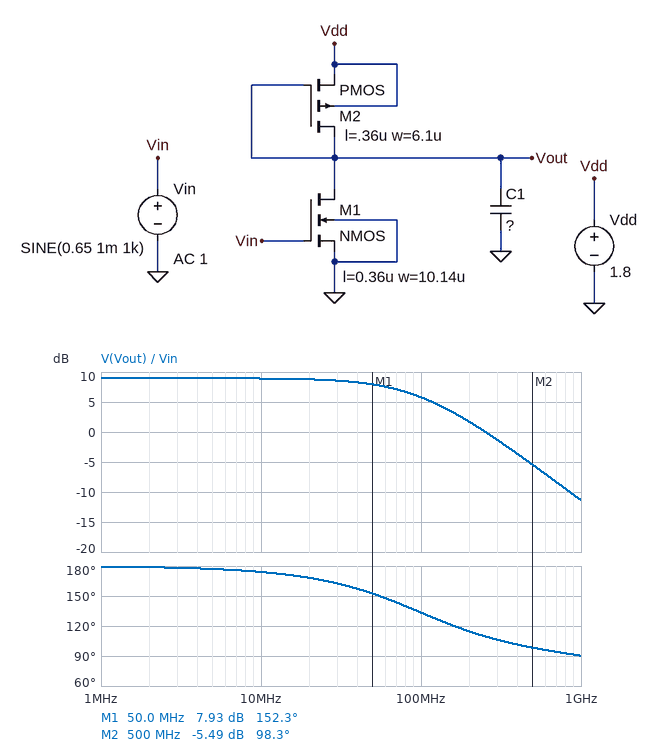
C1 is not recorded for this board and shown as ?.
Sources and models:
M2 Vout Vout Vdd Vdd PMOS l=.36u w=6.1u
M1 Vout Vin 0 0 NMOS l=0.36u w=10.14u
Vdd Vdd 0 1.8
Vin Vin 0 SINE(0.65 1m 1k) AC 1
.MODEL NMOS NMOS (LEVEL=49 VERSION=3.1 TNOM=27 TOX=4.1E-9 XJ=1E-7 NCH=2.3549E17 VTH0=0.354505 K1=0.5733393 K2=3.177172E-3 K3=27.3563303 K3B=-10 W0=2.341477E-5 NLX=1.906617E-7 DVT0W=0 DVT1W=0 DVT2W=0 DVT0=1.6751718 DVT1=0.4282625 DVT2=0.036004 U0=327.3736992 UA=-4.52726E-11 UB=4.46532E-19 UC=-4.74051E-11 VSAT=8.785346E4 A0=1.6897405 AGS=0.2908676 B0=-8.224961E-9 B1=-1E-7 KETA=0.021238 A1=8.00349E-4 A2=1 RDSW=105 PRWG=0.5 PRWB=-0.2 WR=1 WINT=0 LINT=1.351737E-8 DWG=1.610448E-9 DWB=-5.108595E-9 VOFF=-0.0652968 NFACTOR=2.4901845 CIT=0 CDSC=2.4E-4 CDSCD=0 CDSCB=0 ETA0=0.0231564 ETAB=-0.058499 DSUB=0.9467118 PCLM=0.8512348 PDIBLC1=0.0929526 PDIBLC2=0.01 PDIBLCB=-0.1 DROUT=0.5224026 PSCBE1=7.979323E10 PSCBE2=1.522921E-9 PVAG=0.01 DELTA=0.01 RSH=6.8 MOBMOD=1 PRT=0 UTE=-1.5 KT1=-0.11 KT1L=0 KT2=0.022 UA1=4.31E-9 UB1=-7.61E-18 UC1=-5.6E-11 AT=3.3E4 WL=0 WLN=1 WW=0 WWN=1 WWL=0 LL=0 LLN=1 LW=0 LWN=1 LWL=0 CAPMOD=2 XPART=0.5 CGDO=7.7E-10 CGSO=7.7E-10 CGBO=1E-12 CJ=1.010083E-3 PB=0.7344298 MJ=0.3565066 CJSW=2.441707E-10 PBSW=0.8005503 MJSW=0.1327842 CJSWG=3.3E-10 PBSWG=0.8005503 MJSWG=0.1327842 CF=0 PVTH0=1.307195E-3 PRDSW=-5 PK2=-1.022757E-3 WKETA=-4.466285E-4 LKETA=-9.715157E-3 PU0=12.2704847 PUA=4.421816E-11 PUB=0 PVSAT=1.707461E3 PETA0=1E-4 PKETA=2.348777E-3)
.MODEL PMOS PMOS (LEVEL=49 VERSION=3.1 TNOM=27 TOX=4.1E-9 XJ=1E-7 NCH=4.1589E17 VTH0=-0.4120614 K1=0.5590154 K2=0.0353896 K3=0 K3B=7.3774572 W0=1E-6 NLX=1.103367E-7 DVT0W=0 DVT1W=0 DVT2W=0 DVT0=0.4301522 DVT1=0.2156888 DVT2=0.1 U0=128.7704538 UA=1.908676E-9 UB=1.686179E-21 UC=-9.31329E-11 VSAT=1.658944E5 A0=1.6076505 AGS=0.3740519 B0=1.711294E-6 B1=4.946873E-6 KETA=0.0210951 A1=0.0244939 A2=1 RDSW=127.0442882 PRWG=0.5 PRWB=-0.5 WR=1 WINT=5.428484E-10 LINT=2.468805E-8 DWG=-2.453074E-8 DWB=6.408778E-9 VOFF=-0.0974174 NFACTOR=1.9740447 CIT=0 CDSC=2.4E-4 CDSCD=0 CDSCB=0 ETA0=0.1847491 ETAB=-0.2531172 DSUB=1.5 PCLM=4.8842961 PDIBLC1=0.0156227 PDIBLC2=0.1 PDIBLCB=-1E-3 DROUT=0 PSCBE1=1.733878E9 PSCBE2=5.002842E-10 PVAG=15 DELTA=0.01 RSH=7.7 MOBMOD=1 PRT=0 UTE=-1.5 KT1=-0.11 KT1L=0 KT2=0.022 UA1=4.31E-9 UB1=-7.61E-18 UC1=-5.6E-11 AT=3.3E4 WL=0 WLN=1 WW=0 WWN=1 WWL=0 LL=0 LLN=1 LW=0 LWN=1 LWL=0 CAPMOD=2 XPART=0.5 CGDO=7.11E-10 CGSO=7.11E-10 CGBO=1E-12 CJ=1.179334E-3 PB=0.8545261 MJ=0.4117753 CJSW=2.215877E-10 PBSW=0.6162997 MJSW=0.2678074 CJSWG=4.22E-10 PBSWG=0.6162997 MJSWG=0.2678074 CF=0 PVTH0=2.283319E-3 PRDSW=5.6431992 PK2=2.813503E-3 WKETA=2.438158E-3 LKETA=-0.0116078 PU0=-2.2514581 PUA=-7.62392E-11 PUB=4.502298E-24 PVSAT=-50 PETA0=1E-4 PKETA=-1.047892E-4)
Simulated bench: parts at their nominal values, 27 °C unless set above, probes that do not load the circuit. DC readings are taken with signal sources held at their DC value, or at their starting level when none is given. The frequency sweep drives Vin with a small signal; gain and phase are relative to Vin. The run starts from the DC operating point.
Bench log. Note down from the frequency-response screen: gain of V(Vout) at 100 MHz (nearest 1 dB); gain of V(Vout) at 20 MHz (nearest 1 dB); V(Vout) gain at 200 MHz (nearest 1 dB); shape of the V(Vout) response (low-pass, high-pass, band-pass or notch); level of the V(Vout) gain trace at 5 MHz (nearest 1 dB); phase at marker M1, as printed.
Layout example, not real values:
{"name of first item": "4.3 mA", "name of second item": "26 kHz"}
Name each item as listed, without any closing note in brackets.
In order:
{"gain of V(Vout) at 100 MHz": "6 dB", "gain of V(Vout) at 20 MHz": "9 dB", "V(Vout) gain at 200 MHz": "2 dB", "shape of the V(Vout) response": "low-pass", "level of the V(Vout) gain trace at 5 MHz": "9 dB", "phase at marker M1, as printed": "152.3 deg"}
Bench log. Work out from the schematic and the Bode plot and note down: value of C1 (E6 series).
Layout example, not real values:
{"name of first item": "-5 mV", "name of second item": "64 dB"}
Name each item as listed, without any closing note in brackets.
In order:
{"value of C1": "680 fF"}
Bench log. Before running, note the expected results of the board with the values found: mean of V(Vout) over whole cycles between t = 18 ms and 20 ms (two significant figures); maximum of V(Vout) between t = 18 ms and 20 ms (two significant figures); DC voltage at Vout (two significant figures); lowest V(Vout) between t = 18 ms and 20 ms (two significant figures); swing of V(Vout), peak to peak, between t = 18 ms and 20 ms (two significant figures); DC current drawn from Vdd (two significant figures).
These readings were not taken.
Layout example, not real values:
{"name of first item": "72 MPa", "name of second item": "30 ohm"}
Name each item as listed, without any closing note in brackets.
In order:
{"mean of V(Vout) over whole cycles between t = 18 ms and 20 ms": "900 mV", "maximum of V(Vout) between t = 18 ms and 20 ms": "900 mV", "DC voltage at Vout": "900 mV", "lowest V(Vout) between t = 18 ms and 20 ms": "900 mV", "swing of V(Vout), peak to peak, between t = 18 ms and 20 ms": "5.6 mV", "DC current drawn from Vdd": "99 µA"}
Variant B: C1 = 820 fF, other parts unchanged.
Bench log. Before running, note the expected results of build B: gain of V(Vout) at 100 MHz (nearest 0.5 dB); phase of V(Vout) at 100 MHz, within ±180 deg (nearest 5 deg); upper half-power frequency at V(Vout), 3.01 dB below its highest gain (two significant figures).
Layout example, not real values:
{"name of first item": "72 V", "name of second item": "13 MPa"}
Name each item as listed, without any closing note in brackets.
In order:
{"gain of V(Vout) at 100 MHz": "5.0 dB", "phase of V(Vout) at 100 MHz, within ±180 deg": "130 deg", "upper half-power frequency at V(Vout), 3.01 dB below its highest gain": "80 MHz"}
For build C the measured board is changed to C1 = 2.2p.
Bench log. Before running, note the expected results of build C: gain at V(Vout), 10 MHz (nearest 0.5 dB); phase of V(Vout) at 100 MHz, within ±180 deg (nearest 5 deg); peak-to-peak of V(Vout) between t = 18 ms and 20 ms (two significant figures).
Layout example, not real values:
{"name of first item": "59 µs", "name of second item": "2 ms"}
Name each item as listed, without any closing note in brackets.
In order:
{"gain at V(Vout), 10 MHz": "8.5 dB", "phase of V(Vout) at 100 MHz, within ±180 deg": "105 deg", "peak-to-peak of V(Vout) between t = 18 ms and 20 ms": "5.6 mV"}
